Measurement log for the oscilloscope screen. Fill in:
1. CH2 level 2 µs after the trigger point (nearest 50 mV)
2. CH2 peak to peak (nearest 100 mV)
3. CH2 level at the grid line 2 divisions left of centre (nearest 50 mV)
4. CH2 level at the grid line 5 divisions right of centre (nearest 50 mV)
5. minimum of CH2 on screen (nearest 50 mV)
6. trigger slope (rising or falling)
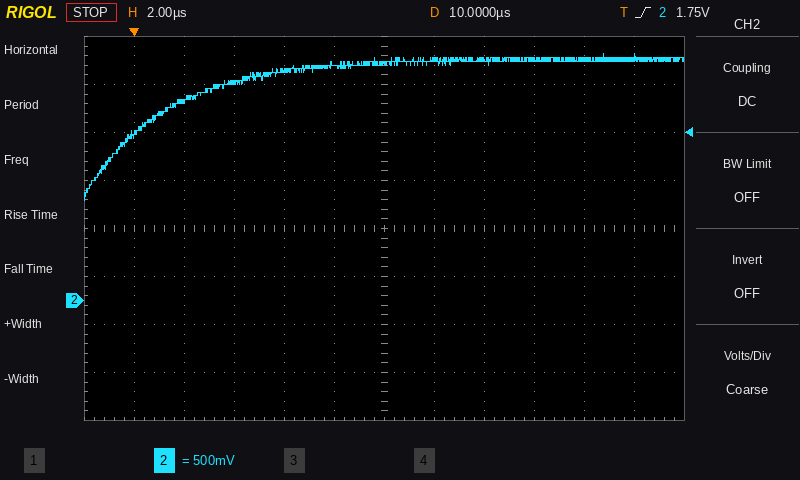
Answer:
2.10 V
1.50 V
2.40 V
2.55 V
1.05 V
rising
